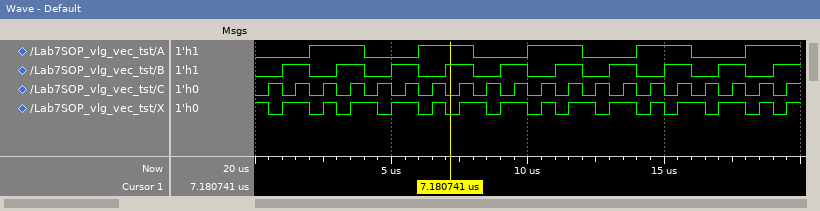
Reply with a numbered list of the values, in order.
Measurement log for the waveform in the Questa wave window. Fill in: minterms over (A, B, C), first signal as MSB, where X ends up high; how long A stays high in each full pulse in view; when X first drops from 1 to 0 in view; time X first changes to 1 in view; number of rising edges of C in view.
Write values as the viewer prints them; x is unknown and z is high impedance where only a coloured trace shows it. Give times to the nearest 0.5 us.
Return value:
1. 0, 2, 3, 5, 7
2. 2 us, 2 us, 2 us, 2 us
3. 0.5 us
4. 1 us
5. 20
